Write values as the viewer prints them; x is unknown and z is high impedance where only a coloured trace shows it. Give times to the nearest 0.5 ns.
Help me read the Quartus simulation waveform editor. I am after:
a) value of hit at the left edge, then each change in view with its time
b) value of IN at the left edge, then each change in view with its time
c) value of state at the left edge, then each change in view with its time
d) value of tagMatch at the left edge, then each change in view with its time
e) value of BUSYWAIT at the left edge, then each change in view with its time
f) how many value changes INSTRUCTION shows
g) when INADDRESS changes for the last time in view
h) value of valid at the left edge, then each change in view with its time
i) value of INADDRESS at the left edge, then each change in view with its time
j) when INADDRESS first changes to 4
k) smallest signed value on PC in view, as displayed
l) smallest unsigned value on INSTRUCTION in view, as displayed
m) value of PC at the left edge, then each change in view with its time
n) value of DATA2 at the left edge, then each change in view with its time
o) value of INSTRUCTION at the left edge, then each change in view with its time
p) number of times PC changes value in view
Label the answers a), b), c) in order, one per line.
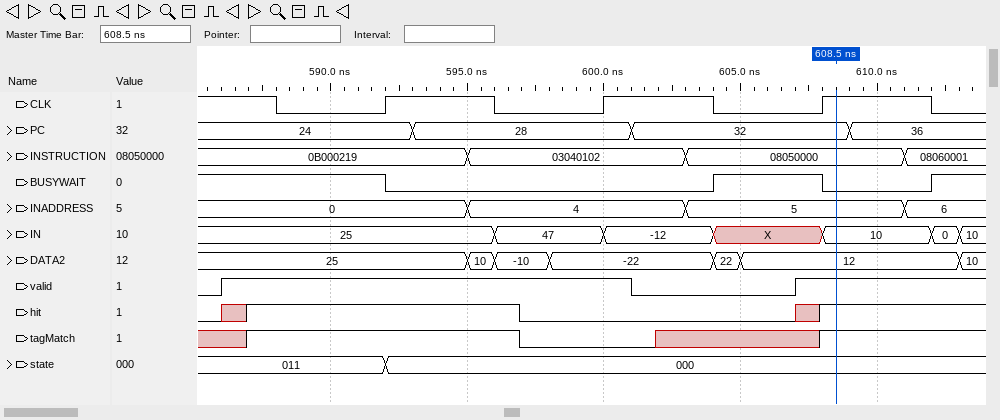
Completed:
a) 0, x at 586 ns, 1 at 587 ns, 0 at 597 ns, x at 607 ns, 1 at 608 ns
b) 25, 47 at 596 ns, -12 at 600 ns, X at 604 ns, 10 at 608 ns, 0 at 612 ns, 10 at 613 ns
c) 011, 000 at 592 ns
d) x, 1 at 587 ns, 0 at 597 ns, x at 602 ns, 1 at 608 ns
e) 1, 0 at 592 ns, 1 at 604 ns, 0 at 608 ns, 1 at 612 ns
f) 3
g) 611 ns
h) 0, 1 at 586 ns, 0 at 601 ns, 1 at 607 ns
i) 0, 4 at 595 ns, 5 at 603 ns, 6 at 611 ns
j) 595 ns
k) 24
l) 03040102
m) 24, 28 at 593 ns, 32 at 601 ns, 36 at 609 ns
n) 25, 10 at 595 ns, -10 at 596 ns, -22 at 598 ns, 22 at 604 ns, 12 at 605 ns, 10 at 613 ns
o) 0B000219, 03040102 at 595 ns, 08050000 at 603 ns, 08060001 at 611 ns
p) 3
